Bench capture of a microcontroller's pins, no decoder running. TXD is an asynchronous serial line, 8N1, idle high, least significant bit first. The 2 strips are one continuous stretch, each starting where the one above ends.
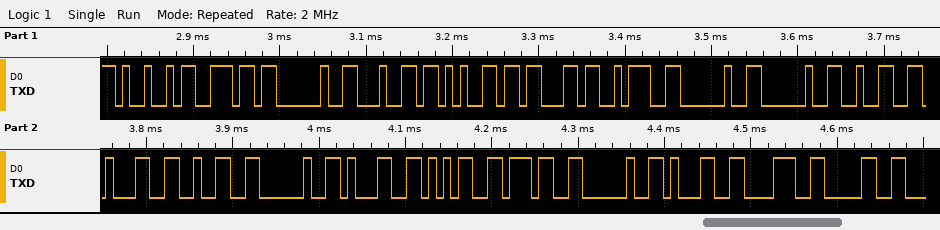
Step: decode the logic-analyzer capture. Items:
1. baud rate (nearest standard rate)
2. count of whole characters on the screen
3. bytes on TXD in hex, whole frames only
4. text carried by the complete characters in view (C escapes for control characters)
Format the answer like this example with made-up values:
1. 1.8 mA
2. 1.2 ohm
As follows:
1. 115200 baud
2. 20
3. 49 6E 20 64 65 63 3A 20 20 32 31 32 20 31 35 37 20 31 38 30
4. "In dec:  212 157 180"
